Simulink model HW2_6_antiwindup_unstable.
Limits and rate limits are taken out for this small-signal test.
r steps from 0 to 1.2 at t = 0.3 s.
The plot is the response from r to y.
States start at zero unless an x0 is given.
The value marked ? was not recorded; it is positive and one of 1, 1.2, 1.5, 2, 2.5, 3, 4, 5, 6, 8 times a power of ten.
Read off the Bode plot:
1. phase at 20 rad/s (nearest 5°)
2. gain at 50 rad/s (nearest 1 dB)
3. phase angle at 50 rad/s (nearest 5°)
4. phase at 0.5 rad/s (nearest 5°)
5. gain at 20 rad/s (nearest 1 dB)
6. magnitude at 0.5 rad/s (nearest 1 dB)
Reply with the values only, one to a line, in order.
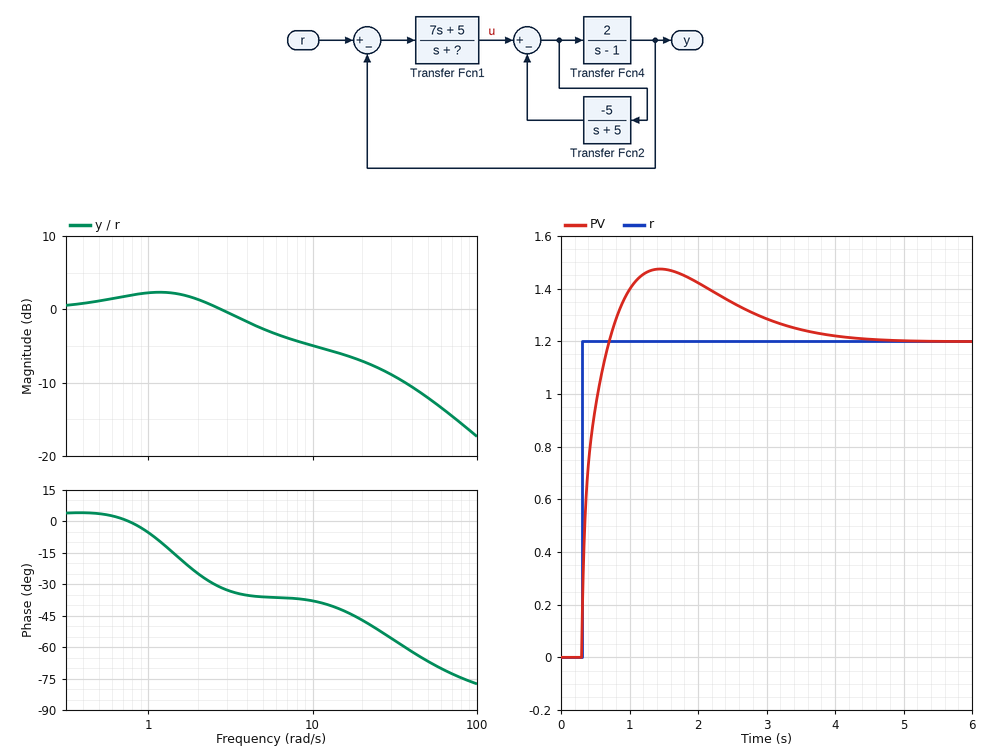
-45°
-12 dB
-65°
5°
-7 dB
1 dB
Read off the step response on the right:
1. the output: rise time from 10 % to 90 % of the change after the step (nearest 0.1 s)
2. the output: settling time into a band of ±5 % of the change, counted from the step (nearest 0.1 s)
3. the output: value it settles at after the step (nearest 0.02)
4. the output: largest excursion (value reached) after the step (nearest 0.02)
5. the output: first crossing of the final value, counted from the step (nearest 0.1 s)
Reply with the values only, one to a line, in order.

0.3 s
3.0 s
1.20
1.48
0.4 s
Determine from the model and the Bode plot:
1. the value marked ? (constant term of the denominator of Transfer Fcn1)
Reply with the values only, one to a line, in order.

15
